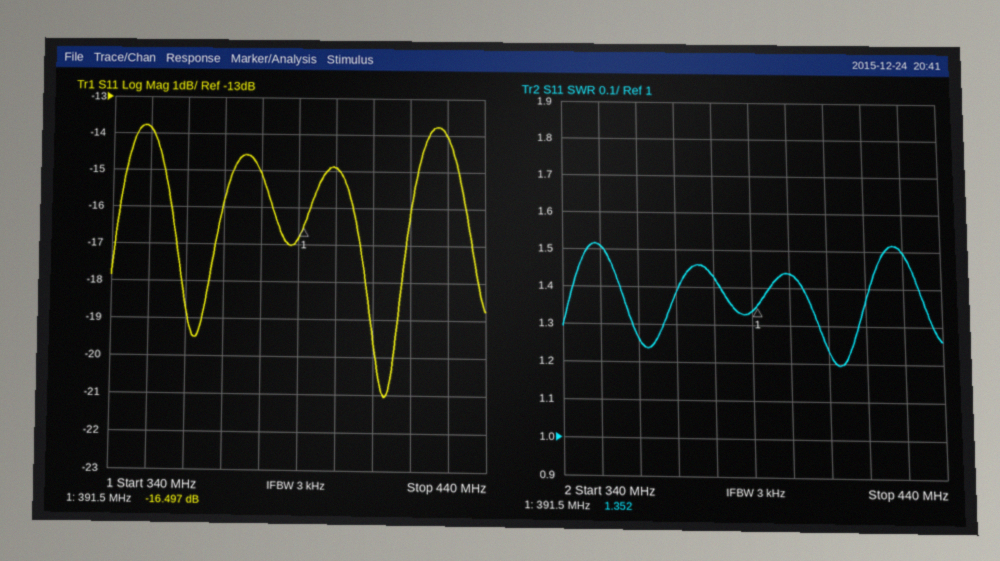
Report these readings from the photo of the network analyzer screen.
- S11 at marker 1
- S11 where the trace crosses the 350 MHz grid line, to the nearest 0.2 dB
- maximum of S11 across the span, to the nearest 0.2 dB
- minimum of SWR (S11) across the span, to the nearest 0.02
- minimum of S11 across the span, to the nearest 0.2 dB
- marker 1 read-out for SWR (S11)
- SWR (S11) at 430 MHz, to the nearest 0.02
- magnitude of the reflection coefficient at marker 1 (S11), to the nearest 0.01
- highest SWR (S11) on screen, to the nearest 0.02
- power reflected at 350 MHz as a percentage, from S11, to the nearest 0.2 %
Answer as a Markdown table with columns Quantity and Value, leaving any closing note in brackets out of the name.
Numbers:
| Quantity | Value |
|---|---|
| S11 at marker 1 | -16.497 dB |
| S11 where the trace crosses the 350 MHz grid line, to the nearest 0.2 dB | -13.8 dB |
| maximum of S11 across the span, to the nearest 0.2 dB | -13.8 dB |
| minimum of SWR (S11) across the span, to the nearest 0.02 | 1.20 |
| minimum of S11 across the span, to the nearest 0.2 dB | -21.0 dB |
| marker 1 read-out for SWR | 1.352 |
| SWR (S11) at 430 MHz, to the nearest 0.02 | 1.50 |
| magnitude of the reflection coefficient at marker 1 (S11), to the nearest 0.01 | 0.15 |
| highest SWR (S11) on screen, to the nearest 0.02 | 1.52 |
| power reflected at 350 MHz as a percentage, from S11, to the nearest 0.2 % | 4.2 % |
